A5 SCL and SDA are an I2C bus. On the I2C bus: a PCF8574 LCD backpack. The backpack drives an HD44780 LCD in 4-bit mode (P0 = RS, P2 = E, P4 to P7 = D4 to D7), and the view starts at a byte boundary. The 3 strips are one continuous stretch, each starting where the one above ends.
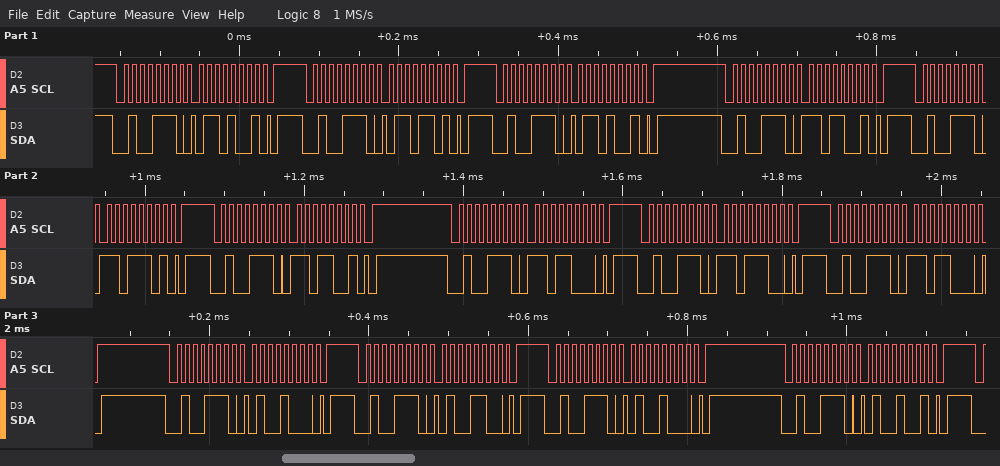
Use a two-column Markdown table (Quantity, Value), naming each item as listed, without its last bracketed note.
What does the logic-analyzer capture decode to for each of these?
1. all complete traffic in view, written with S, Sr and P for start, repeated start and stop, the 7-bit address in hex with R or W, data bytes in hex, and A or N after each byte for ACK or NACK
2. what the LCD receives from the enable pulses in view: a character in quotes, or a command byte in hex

| Quantity | Value |
|---|---|
| all complete traffic in view, written with S, Sr and P for start, repeated start and stop, the 7-bit address in hex with R or W, data bytes in hex, and A or N after each byte for ACK or NACK | S 27W A 69 A P S 27W A 6D A P S 27W A 69 A P S 27W A D9 A P S 27W A DD A P S 27W A D9 A P S 27W A D8 A P S 27W A DC A P S 27W A D8 A P S 27W A 48 A P S 27W A 4C A P S 27W A 48 A P S 27W A 49 A P |
| what the LCD receives from the enable pulses in view: a character in quotes, or a command byte in hex | 'm' 0xD4 |
